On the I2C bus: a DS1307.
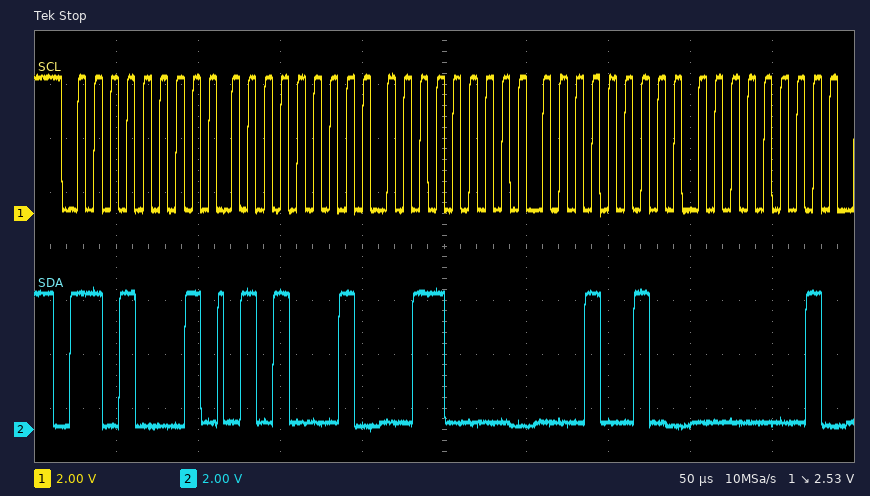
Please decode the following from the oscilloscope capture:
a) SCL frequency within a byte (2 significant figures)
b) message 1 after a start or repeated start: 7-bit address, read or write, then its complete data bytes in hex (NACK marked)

100 kHz
0x68 read: 51 30 12 01
